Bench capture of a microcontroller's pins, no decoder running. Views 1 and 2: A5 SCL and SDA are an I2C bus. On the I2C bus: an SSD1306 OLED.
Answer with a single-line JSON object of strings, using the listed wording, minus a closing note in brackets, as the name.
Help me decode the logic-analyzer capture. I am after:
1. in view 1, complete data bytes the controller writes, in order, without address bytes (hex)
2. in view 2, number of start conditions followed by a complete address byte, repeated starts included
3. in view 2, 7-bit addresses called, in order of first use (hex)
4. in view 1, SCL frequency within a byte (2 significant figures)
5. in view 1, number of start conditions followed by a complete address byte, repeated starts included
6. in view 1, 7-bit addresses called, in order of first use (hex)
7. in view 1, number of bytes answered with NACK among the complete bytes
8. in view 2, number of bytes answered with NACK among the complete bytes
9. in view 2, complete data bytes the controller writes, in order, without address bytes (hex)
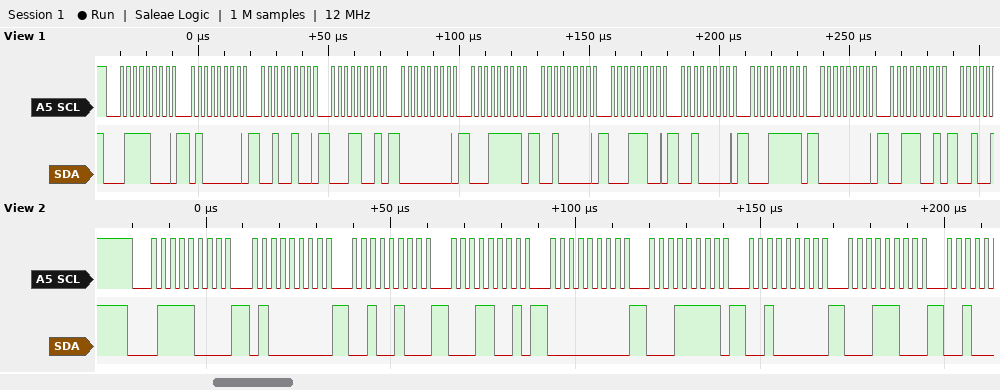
{"in view 1, complete data bytes the controller writes, in order, without address bytes": "40 24 19 00 1F 20 1C 20 1F 00 39", "in view 2, number of start conditions followed by a complete address byte, repeated starts included": "1", "in view 2, 7-bit addresses called, in order of first use": "0x3C", "in view 1, SCL frequency within a byte": "400 kHz", "in view 1, number of start conditions followed by a complete address byte, repeated starts included": "1", "in view 1, 7-bit addresses called, in order of first use": "0x3C", "in view 1, number of bytes answered with NACK among the complete bytes": "0", "in view 2, number of bytes answered with NACK among the complete bytes": "0", "in view 2, complete data bytes the controller writes, in order, without address bytes": "40 24 19 00 1F 20 1C"}
